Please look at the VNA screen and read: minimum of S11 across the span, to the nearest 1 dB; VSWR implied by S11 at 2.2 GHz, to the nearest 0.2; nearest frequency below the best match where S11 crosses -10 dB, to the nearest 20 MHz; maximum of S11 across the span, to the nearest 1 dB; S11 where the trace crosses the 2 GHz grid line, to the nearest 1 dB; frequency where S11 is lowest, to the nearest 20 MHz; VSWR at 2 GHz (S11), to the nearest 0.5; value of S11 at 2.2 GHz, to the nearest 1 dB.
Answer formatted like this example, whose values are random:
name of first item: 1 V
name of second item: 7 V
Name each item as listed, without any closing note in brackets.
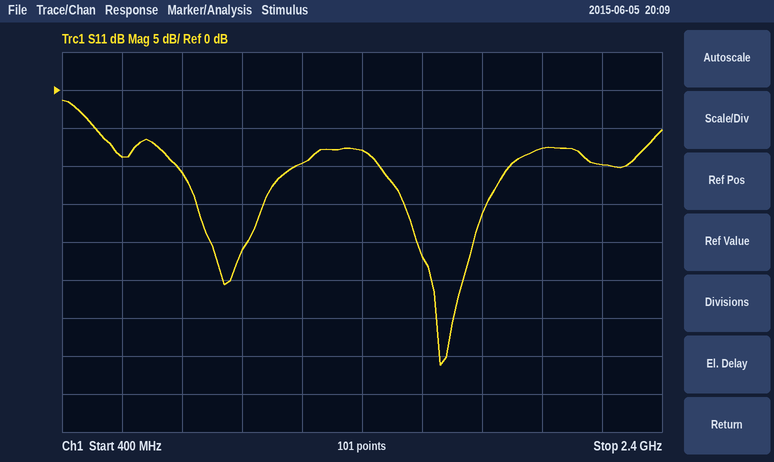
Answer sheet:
minimum of S11 across the span, to the nearest 1 dB: -36 dB
VSWR implied by S11 at 2.2 GHz, to the nearest 0.2: 2.0
nearest frequency below the best match where S11 crosses -10 dB, to the nearest 20 MHz: 1.46 GHz
maximum of S11 across the span, to the nearest 1 dB: -1 dB
S11 where the trace crosses the 2 GHz grid line, to the nearest 1 dB: -8 dB
frequency where S11 is lowest, to the nearest 20 MHz: 1.66 GHz
VSWR at 2 GHz (S11), to the nearest 0.5: 2.5
value of S11 at 2.2 GHz, to the nearest 1 dB: -10 dB
